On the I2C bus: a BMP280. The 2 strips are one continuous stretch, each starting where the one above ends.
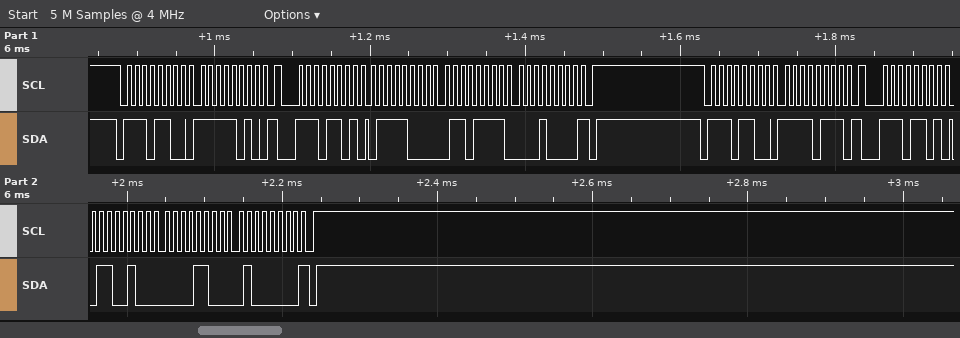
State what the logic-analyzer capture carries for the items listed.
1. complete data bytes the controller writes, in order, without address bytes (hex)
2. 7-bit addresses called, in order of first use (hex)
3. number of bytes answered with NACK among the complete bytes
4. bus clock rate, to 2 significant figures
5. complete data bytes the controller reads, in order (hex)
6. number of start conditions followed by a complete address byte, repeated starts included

FA F7
0x76
2
100 kHz
78 6F 10 64 0C 40
4
